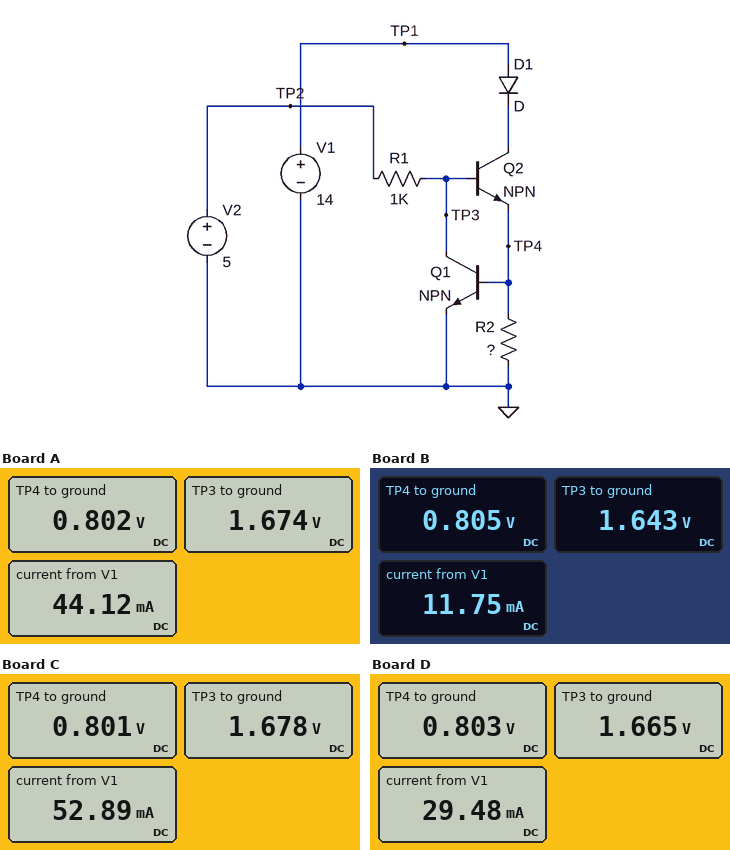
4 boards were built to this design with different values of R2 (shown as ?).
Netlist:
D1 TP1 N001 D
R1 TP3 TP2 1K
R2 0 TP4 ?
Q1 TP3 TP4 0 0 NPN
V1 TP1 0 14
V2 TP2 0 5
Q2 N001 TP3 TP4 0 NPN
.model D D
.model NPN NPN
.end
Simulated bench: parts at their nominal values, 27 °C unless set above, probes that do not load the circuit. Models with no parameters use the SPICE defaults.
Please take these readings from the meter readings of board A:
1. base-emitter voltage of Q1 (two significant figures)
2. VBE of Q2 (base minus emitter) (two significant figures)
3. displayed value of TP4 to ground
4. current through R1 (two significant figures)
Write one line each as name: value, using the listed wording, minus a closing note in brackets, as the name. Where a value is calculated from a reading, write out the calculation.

base-emitter voltage of Q1: 802 mV = 800 mV
VBE of Q2 (base minus emitter): 1.674 V - 802 mV = 870 mV
displayed value of TP4 to ground: 0.802 V
current through R1: (5 V - 1.674 V) / 1 kΩ = 3.3 mA
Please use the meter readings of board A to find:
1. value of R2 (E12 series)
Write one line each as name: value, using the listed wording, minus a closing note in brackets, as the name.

value of R2: 18 Ω
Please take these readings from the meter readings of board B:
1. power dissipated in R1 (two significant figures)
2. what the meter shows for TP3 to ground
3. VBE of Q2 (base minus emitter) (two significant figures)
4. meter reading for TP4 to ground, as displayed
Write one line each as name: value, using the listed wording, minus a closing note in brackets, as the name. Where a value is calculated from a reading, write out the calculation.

power dissipated in R1: (5 V - 1.643 V)^2 / 1 kΩ = 11 mW
what the meter shows for TP3 to ground: 1.643 V
VBE of Q2 (base minus emitter): 1.643 V - 805 mV = 840 mV
meter reading for TP4 to ground, as displayed: 0.805 V
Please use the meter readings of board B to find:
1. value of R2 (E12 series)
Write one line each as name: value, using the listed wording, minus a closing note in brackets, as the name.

value of R2: 68 Ω
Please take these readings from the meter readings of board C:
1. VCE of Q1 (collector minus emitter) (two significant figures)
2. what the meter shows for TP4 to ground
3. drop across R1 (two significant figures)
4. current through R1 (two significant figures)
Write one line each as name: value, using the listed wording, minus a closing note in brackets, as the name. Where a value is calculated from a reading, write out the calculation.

VCE of Q1 (collector minus emitter): 1.678 V = 1.7 V
what the meter shows for TP4 to ground: 0.801 V
drop across R1: 5 V - 1.678 V = 3.3 V
current through R1: (5 V - 1.678 V) / 1 kΩ = 3.3 mA
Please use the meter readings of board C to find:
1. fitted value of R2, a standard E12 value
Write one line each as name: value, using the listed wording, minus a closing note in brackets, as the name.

fitted value of R2, a standard E12 value: 15 Ω
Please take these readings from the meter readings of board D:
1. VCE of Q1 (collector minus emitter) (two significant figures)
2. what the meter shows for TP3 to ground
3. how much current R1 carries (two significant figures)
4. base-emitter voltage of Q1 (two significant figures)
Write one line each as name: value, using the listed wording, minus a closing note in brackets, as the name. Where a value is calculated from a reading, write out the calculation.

VCE of Q1 (collector minus emitter): 1.665 V = 1.7 V
what the meter shows for TP3 to ground: 1.665 V
how much current R1 carries: (5 V - 1.665 V) / 1 kΩ = 3.3 mA
base-emitter voltage of Q1: 803 mV = 800 mV
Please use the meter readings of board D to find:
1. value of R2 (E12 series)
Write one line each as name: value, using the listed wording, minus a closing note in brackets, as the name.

value of R2: 27 Ω
